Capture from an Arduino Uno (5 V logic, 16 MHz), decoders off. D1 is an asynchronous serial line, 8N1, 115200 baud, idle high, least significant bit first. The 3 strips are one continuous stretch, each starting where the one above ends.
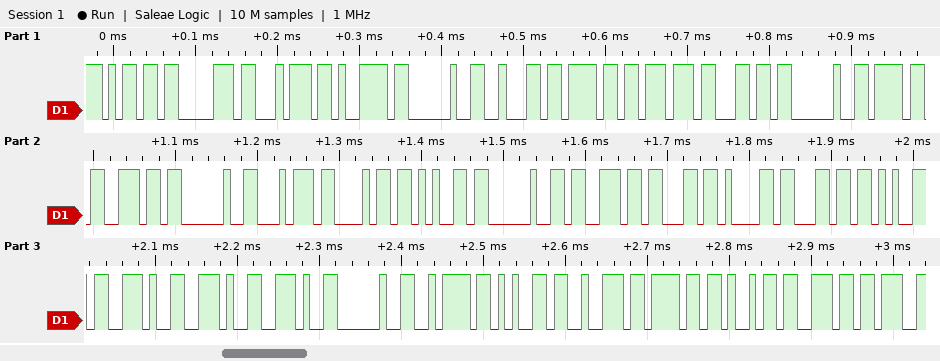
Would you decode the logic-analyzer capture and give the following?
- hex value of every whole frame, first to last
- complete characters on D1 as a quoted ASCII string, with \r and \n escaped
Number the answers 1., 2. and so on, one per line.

1. 6D 70 74 79 20 62 6F 77 6C 20 6F 6E 20 74 68 65 20 73 63 61 6C 65 2E 2E 2E 20 7A 65 72 6F 69 6E
2. "mpty bowl on the scale... zeroin"
